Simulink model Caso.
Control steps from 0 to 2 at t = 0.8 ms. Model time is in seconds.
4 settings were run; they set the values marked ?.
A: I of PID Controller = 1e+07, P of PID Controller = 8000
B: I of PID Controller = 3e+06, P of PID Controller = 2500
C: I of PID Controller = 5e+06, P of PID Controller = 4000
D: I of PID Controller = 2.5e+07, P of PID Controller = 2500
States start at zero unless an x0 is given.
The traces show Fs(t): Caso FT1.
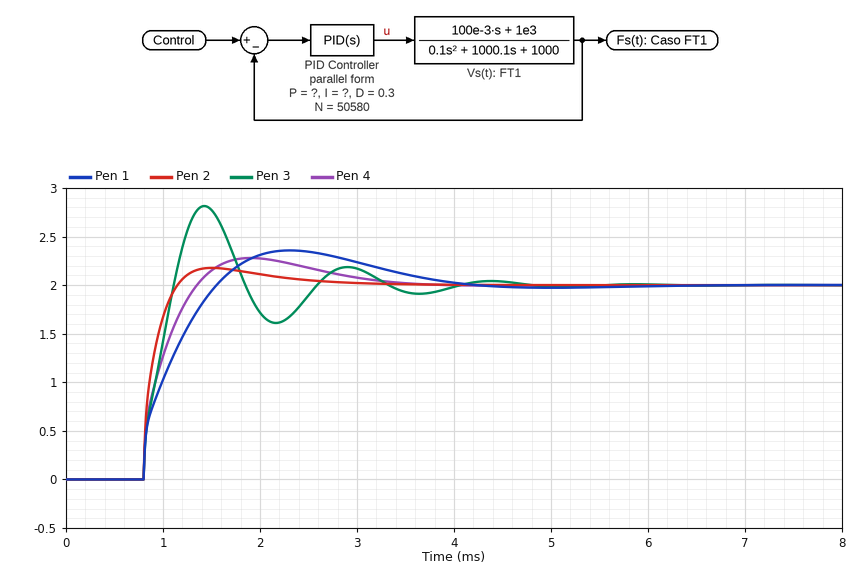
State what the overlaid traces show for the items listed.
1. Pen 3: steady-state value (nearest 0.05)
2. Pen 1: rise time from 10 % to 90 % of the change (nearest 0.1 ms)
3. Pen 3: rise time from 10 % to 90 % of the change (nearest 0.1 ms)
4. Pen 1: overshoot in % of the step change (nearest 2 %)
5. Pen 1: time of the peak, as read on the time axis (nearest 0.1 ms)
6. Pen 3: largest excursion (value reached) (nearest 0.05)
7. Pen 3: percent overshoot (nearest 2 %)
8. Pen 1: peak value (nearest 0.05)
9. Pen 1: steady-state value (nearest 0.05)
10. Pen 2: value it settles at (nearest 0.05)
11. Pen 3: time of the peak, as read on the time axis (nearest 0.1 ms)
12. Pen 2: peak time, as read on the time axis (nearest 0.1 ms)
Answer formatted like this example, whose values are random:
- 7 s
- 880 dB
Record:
- 2.00
- 0.6 ms
- 0.3 ms
- 18 %
- 2.3 ms
- 2.80
- 40 %
- 2.35
- 2.00
- 2.00
- 1.4 ms
- 1.5 ms
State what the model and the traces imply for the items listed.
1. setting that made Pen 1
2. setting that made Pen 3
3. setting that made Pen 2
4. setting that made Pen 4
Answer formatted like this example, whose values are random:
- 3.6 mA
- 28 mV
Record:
- B
- D
- A
- C
